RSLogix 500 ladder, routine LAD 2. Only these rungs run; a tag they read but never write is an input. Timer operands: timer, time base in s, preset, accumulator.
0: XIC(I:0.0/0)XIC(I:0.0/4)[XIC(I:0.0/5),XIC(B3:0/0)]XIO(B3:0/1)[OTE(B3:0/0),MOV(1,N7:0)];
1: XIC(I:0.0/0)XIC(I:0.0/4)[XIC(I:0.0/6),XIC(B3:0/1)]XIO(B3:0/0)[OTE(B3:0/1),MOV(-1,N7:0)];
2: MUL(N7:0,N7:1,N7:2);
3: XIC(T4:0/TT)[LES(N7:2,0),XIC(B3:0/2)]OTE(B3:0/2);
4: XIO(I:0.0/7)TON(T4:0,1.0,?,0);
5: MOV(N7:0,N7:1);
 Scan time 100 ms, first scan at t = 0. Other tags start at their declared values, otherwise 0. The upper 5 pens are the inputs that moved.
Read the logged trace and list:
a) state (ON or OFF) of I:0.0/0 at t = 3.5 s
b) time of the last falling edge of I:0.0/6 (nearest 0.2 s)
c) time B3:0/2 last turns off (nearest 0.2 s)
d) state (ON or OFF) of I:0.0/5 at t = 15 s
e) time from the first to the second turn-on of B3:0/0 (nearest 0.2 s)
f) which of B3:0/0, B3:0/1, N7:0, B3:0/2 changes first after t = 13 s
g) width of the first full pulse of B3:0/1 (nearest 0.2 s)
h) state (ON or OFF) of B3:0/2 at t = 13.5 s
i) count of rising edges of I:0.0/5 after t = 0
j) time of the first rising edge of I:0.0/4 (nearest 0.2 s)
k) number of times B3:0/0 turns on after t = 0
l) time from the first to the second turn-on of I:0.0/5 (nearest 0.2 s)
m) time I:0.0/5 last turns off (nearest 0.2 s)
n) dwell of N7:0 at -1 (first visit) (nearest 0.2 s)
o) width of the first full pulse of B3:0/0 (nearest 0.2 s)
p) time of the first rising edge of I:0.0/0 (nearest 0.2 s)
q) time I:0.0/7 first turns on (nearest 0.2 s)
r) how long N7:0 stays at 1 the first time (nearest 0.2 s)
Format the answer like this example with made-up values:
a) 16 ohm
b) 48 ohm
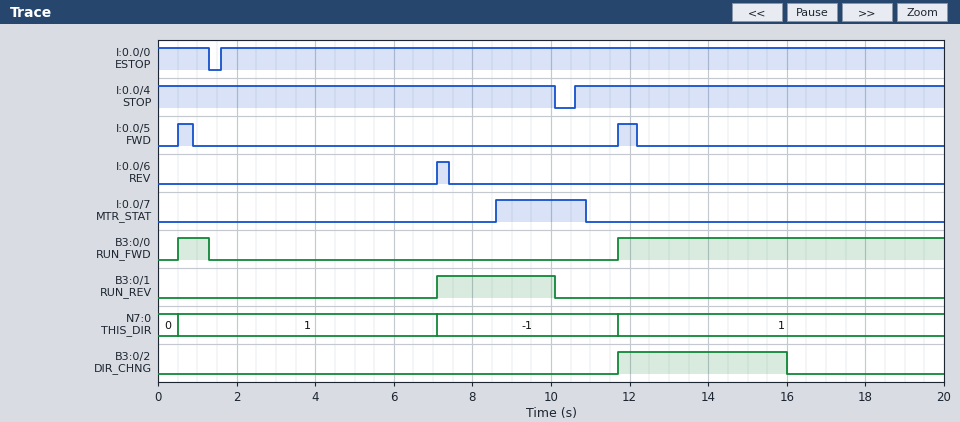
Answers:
a) ON
b) 7.4 s
c) 16.0 s
d) OFF
e) 11.2 s
f) B3:0/2
g) 3.0 s
h) ON
i) 2
j) 10.6 s
k) 2
l) 11.2 s
m) 12.2 s
n) 4.6 s
o) 0.8 s
p) 1.6 s
q) 8.6 s
r) 6.6 s
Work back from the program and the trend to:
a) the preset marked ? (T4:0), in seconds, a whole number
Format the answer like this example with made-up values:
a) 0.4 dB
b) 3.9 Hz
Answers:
a) 5 s
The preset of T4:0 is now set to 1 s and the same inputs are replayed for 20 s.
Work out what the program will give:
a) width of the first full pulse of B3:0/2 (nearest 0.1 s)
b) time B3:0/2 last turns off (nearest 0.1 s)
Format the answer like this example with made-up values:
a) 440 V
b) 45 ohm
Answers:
a) 0.3 s
b) 12.0 s
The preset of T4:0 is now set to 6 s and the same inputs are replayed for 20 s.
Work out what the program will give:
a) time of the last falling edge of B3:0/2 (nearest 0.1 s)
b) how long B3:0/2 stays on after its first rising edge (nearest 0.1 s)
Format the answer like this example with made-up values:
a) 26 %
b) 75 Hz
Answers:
a) 17.0 s
b) 5.3 s
